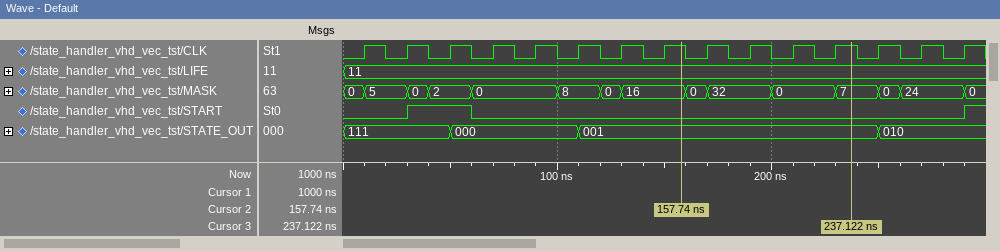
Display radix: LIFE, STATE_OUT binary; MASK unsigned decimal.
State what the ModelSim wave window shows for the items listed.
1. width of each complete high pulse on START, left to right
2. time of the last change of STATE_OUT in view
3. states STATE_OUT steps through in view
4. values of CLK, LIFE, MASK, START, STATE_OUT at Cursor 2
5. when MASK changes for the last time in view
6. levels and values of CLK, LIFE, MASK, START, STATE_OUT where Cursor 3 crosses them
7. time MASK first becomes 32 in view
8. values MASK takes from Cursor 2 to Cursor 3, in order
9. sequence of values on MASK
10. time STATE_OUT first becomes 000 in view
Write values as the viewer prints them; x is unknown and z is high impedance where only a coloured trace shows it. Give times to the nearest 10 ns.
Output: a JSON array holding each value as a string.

["30 ns", "250 ns", "111, 000, 001, 010", "CLK=1, LIFE=11, MASK=16, START=0, STATE_OUT=001", "290 ns", "CLK=1, LIFE=11, MASK=7, START=0, STATE_OUT=001", "170 ns", "16, 0, 32, 0, 7", "0, 5, 0, 2, 0, 8, 0, 16, 0, 32, 0, 7, 0, 24, 0", "50 ns"]
